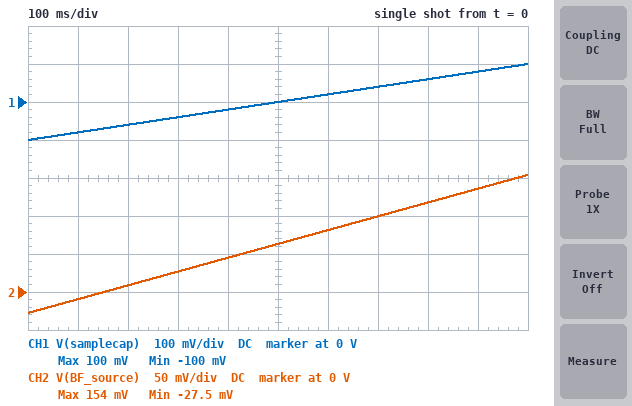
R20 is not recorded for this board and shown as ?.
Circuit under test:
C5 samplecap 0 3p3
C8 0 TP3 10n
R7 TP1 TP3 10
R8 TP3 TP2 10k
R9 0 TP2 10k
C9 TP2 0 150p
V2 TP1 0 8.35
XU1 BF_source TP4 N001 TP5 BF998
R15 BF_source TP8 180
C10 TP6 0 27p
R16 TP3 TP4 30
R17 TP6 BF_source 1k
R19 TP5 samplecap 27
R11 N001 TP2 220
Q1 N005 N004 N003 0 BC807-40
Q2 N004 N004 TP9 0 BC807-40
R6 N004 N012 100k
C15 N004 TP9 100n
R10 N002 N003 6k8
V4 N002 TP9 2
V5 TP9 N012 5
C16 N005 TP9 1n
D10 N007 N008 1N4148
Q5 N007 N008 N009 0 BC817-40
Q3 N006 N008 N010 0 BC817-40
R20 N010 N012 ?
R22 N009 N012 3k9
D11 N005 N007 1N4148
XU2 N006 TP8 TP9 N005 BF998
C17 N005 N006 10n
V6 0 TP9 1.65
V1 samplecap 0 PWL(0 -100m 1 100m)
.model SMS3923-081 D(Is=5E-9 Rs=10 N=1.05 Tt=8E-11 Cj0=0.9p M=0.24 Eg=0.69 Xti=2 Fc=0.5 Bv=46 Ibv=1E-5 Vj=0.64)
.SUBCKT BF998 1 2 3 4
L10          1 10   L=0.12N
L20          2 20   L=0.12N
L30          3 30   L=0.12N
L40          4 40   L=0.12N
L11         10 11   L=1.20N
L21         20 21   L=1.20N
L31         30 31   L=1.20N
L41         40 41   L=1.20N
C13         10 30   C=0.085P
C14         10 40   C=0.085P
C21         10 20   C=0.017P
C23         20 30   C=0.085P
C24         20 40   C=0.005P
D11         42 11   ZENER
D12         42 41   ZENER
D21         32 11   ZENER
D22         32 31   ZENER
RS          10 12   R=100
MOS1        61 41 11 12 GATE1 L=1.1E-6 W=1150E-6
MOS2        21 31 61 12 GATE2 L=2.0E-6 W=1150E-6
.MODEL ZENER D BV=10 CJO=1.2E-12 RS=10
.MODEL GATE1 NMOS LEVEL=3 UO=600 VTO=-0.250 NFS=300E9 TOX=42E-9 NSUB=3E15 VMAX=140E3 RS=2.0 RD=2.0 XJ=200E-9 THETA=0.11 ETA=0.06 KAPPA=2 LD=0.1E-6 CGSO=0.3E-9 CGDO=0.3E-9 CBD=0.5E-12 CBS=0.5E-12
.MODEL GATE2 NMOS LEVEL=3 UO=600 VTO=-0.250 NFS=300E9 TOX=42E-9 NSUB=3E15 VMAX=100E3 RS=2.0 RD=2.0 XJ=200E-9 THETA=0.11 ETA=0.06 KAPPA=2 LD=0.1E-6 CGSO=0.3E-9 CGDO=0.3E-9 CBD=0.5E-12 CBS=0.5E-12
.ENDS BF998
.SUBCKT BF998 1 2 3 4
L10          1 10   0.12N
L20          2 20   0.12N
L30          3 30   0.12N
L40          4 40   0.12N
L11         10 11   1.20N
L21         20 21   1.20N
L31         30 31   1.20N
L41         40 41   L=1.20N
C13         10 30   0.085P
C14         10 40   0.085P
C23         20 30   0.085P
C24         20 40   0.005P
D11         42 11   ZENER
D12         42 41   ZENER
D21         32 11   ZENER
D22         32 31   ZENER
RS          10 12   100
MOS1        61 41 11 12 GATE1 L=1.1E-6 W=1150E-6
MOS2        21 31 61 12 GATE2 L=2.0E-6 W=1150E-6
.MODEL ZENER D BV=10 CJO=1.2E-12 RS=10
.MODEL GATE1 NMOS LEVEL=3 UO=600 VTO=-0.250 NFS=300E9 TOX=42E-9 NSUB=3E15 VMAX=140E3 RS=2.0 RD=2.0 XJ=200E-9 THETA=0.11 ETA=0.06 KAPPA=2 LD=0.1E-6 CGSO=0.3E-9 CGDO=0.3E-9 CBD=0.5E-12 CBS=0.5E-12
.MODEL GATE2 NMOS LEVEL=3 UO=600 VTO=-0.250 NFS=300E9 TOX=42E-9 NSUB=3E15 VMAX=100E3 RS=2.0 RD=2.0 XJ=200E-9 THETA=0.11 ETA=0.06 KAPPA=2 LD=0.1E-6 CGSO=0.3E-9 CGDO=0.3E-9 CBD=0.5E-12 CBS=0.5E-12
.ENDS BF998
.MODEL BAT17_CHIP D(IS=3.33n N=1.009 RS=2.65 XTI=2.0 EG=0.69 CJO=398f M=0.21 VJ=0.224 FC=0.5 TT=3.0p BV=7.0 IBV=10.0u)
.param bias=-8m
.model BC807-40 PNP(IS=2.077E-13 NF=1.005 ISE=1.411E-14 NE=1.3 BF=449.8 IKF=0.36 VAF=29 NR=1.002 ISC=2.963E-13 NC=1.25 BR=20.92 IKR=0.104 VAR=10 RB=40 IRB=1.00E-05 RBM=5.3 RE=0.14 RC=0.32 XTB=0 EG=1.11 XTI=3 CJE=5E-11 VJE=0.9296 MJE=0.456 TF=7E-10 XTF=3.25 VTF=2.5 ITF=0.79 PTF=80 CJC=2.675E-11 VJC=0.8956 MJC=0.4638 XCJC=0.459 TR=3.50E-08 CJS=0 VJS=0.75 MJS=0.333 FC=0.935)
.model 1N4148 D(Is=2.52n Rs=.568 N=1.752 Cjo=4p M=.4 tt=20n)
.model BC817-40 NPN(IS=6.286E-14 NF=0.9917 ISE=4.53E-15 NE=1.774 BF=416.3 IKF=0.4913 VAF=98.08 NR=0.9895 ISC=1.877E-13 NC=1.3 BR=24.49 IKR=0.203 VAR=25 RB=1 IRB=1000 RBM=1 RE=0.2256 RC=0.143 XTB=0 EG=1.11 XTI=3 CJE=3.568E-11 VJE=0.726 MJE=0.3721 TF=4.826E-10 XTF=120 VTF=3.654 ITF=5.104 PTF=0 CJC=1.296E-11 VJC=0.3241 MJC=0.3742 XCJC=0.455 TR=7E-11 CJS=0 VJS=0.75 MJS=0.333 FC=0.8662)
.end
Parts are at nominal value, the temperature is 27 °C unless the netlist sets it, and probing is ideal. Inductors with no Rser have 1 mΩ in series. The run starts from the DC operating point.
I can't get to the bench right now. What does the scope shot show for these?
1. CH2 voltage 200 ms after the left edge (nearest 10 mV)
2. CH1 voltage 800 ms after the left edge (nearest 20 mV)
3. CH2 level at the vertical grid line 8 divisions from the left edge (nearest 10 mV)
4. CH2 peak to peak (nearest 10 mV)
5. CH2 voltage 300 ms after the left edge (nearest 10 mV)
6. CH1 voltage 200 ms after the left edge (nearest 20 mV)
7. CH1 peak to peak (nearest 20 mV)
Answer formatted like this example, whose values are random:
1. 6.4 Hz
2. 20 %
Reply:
1. 10 mV
2. 60 mV
3. 120 mV
4. 180 mV
5. 30 mV
6. -60 mV
7. 200 mV
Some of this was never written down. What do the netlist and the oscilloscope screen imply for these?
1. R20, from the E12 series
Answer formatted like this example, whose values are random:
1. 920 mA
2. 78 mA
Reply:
1. 120 Ω
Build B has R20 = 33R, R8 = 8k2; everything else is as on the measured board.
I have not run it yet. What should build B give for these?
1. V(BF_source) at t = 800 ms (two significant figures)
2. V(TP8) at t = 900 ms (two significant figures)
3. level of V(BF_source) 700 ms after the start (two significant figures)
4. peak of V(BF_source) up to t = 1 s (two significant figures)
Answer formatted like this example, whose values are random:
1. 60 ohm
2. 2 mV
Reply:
1. -320 mV
2. -4.4 V
3. -340 mV
4. -290 mV
